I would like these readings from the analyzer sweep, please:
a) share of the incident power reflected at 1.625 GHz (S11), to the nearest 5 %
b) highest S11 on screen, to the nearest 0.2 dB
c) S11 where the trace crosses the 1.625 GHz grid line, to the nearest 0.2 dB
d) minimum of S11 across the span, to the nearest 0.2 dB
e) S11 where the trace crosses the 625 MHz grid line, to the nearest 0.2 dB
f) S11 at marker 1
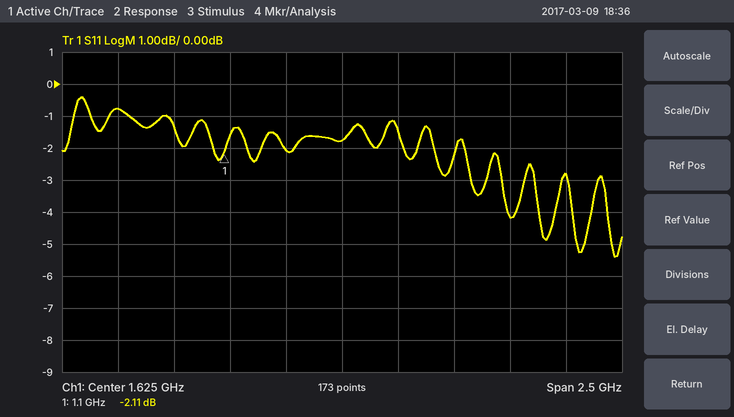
65 %
-0.4 dB
-1.8 dB
-5.4 dB
-0.8 dB
-2.11 dB
